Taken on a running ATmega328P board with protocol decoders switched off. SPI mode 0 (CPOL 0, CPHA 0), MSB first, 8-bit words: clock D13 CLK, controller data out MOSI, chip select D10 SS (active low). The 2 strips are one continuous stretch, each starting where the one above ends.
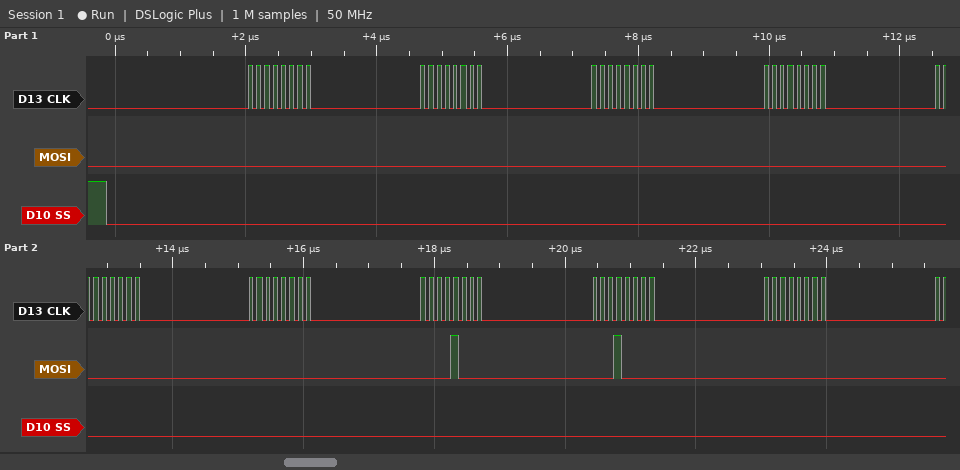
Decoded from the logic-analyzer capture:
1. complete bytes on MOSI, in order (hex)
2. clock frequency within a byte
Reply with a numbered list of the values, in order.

1. 0x00 0x00 0x00 0x00 0x00 0x00 0x08 0x10 0x00
2. 8 MHz
